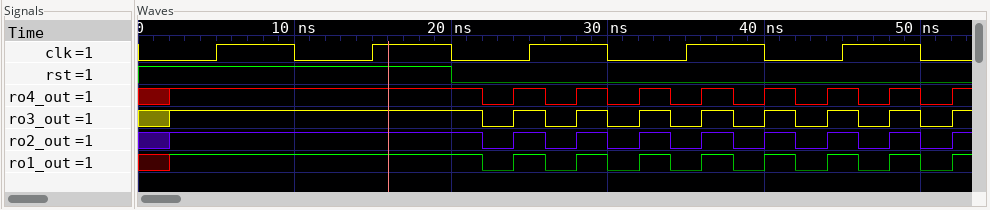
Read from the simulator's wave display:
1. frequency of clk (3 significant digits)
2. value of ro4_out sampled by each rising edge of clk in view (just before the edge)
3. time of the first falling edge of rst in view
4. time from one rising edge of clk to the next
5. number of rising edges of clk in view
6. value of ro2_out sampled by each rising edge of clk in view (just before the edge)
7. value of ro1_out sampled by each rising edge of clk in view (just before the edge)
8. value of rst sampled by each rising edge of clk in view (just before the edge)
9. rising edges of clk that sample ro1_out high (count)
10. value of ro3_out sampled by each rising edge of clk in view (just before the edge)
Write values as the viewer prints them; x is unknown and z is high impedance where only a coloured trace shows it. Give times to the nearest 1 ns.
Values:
100 MHz
1 1 1 0 1
20 ns
10 ns
5
1 1 1 0 1
1 1 1 0 1
1 1 0 0 0
4
1 1 1 0 1
